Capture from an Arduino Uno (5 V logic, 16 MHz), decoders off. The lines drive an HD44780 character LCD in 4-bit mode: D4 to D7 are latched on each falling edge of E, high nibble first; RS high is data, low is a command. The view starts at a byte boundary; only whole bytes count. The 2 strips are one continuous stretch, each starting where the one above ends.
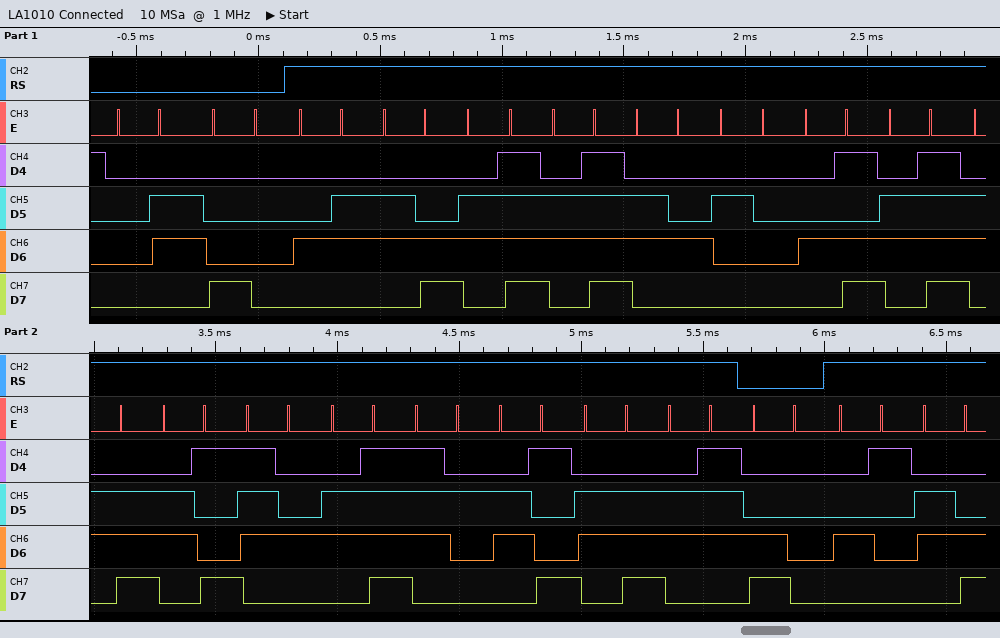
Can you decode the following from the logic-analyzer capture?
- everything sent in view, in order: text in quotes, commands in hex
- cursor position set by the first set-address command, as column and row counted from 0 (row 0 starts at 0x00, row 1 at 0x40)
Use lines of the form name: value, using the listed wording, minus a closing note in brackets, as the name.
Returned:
everything sent in view, in order: text in quotes, commands in hex: 0x06 0x80 "Flood Monitoring" 0xC0 "Al"
cursor position set by the first set-address command, as column and row counted from 0: column 0, row 0
